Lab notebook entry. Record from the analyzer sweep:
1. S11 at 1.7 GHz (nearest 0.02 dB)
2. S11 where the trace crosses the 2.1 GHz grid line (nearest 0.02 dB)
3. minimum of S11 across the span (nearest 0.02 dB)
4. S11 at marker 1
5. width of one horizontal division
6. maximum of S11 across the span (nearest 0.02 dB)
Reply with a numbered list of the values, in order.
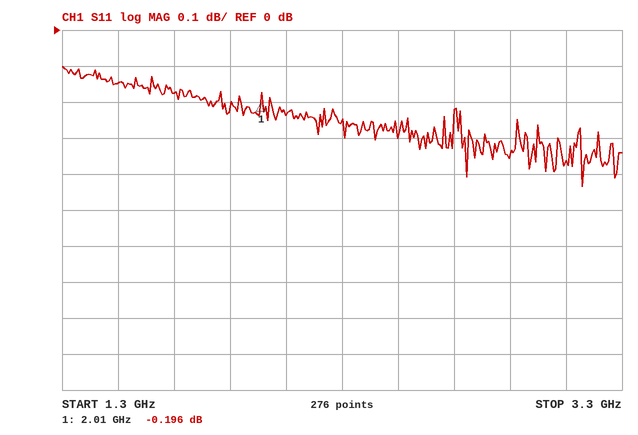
1. -0.18 dB
2. -0.24 dB
3. -0.44 dB
4. -0.196 dB
5. 200 MHz
6. -0.10 dB
